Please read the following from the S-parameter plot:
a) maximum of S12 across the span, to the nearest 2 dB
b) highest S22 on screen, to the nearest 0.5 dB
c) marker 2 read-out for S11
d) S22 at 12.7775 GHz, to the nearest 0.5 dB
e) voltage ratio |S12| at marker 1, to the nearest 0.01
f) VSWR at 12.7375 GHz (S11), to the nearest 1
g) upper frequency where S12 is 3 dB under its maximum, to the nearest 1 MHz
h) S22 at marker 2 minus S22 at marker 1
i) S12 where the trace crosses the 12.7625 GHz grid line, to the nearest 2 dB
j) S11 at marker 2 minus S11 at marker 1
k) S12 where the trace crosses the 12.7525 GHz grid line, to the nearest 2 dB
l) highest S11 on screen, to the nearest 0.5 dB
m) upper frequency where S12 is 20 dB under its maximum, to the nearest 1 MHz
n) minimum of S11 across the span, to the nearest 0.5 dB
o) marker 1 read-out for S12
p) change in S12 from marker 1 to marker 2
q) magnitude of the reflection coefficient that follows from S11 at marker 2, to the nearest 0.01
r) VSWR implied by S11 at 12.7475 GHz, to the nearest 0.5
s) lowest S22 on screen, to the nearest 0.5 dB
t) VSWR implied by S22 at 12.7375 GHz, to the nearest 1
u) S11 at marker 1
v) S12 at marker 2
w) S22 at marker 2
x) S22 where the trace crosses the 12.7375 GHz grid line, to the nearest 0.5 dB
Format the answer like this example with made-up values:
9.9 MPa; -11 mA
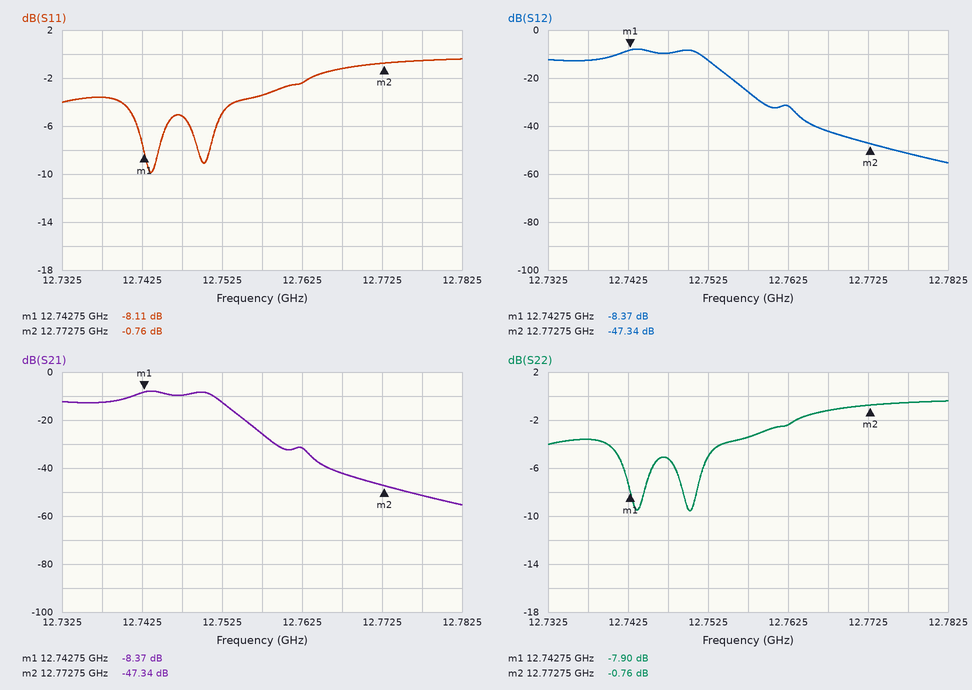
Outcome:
-8 dB; -0.5 dB; -0.76 dB; -0.5 dB; 0.38; 5; 12.752 GHz; 7.14 dB; -32 dB; 7.35 dB; -12 dB; -0.5 dB; 12.758 GHz; -10.0 dB; -8.37 dB; -38.97 dB; 0.92; 3.5; -9.5 dB; 5; -8.11 dB; -47.34 dB; -0.76 dB; -3.5 dB
